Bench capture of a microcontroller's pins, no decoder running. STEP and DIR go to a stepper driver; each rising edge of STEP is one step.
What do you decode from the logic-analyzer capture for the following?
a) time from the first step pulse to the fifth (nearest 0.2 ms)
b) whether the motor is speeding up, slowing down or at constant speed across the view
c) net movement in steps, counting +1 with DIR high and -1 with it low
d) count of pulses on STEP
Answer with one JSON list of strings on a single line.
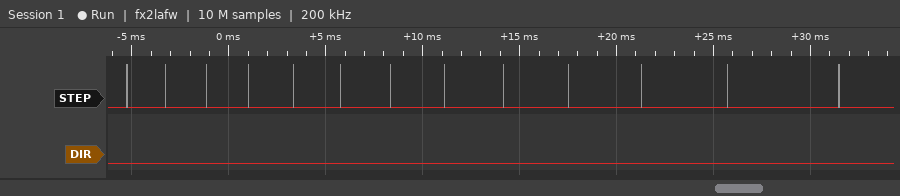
["8.6 ms", "slowing down", "-13", "13"]
